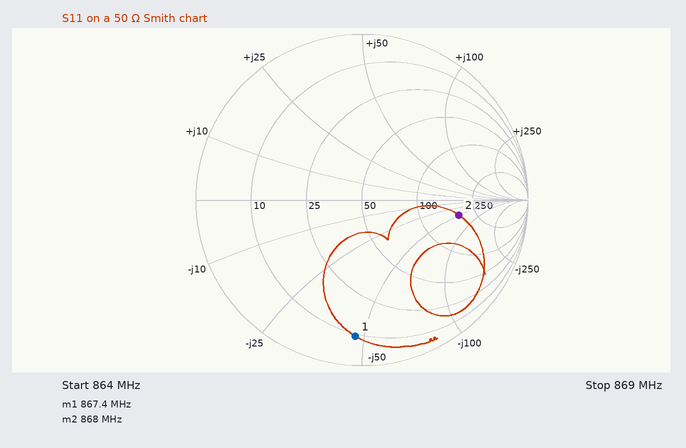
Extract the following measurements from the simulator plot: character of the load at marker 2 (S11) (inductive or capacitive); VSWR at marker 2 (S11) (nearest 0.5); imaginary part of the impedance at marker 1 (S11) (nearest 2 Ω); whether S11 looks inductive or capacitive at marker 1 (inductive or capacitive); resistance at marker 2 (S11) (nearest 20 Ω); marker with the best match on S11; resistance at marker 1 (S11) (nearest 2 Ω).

capacitive
4.0
-46 Ω
capacitive
180 Ω
marker 2
10 Ω
